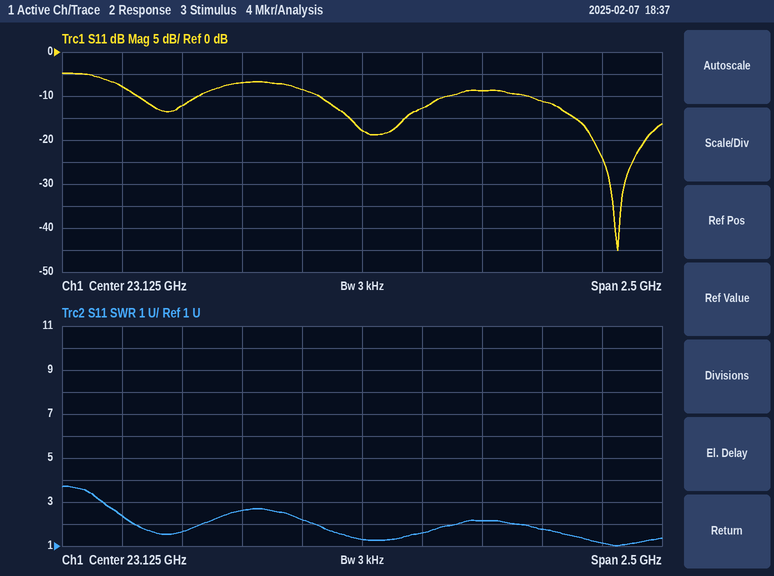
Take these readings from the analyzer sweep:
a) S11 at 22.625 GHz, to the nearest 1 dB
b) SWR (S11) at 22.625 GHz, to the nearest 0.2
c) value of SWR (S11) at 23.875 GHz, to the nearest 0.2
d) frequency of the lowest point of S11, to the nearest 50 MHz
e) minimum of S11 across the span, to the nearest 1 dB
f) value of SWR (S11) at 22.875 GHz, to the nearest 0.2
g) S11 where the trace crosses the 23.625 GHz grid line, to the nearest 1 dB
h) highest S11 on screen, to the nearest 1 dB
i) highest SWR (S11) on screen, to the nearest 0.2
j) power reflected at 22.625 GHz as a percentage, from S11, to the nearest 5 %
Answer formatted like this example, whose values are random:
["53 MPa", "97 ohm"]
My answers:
["-7 dB", "2.6", "1.8", "24.20 GHz", "-45 dB", "2.2", "-9 dB", "-5 dB", "3.8", "20 %"]
